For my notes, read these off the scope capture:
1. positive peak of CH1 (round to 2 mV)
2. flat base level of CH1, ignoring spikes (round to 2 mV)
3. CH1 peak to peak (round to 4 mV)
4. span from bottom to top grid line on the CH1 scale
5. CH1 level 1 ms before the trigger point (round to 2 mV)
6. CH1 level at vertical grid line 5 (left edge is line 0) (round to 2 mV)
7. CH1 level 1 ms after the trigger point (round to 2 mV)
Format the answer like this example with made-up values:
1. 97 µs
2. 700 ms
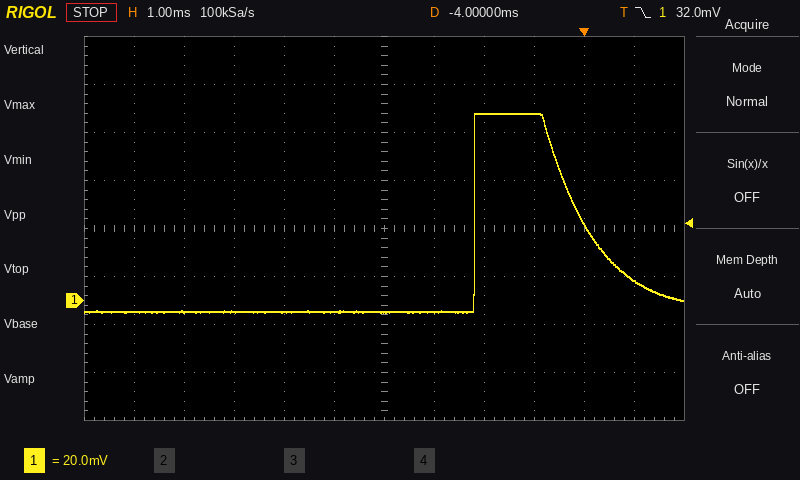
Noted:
1. 78 mV
2. -4 mV
3. 84 mV
4. 160 mV
5. 78 mV
6. -4 mV
7. 8 mV
